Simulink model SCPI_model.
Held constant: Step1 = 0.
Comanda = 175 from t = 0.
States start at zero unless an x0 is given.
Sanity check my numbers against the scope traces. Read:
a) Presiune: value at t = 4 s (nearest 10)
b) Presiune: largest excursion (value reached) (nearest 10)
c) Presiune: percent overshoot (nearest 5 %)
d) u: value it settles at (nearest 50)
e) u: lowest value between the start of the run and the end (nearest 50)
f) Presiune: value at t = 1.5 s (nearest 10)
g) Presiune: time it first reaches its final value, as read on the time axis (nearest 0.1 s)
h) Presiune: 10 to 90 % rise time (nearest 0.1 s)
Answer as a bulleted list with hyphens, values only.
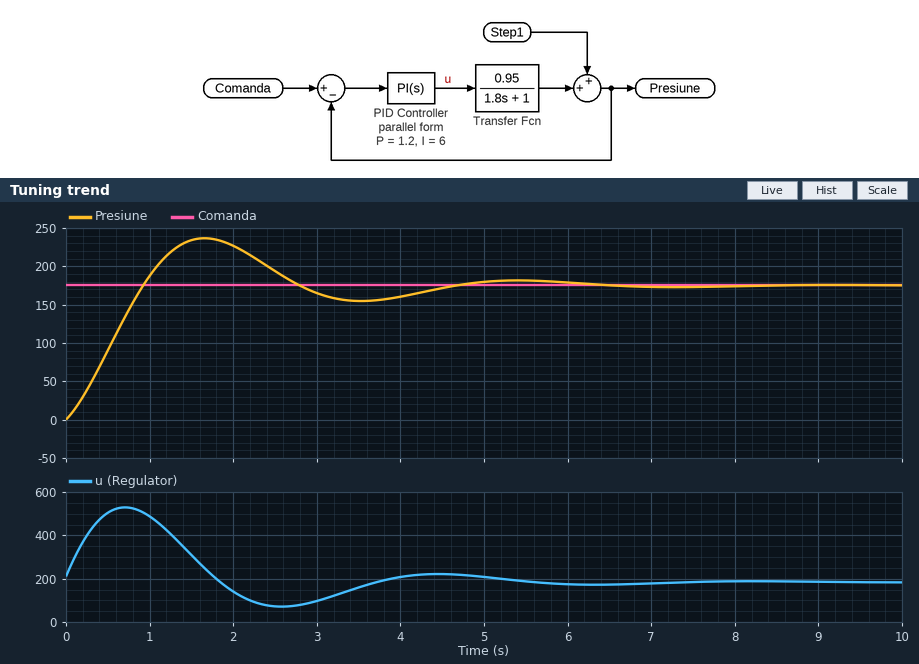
- 160
- 240
- 35 %
- 200
- 50
- 230
- 0.9 s
- 0.7 s
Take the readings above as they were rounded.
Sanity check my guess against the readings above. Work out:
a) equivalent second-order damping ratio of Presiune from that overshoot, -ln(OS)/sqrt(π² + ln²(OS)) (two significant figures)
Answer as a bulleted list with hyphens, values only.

- 0.32
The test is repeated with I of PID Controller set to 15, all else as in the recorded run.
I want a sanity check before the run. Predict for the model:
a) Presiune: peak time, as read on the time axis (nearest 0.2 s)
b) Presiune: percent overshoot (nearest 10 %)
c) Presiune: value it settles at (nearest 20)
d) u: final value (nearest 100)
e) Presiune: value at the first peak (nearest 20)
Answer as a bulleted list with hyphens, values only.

- 1.0 s
- 50 %
- 180
- 200
- 260
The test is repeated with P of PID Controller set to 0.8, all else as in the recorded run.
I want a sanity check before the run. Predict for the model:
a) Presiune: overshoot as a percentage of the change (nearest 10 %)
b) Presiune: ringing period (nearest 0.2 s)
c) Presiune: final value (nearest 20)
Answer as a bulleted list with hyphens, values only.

- 40 %
- 3.6 s
- 180
